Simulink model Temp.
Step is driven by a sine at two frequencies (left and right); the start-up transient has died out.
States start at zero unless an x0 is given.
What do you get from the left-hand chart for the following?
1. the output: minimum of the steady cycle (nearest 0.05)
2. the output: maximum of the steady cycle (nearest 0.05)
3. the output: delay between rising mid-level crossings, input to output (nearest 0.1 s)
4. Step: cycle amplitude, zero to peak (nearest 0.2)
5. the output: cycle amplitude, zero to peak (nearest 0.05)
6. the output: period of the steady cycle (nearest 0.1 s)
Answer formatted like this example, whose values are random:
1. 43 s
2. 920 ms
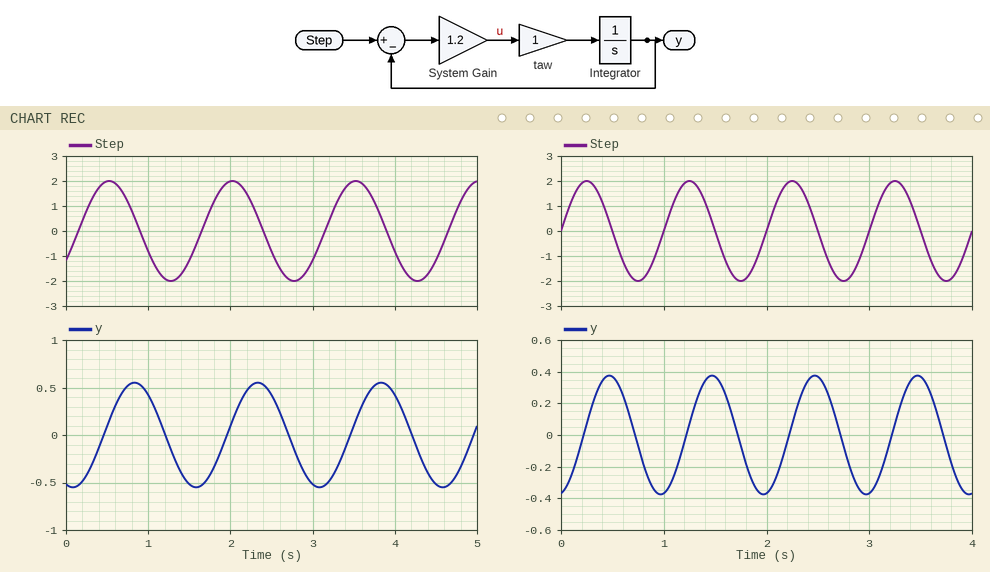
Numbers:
1. -0.55
2. 0.55
3. 0.3 s
4. 2.0
5. 0.55
6. 1.5 s
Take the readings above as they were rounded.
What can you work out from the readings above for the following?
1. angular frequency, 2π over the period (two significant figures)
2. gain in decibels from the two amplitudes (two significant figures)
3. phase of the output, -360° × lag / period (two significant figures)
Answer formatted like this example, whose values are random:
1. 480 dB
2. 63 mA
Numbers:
1. 4.2 rad/s
2. -11 dB
3. -72°
